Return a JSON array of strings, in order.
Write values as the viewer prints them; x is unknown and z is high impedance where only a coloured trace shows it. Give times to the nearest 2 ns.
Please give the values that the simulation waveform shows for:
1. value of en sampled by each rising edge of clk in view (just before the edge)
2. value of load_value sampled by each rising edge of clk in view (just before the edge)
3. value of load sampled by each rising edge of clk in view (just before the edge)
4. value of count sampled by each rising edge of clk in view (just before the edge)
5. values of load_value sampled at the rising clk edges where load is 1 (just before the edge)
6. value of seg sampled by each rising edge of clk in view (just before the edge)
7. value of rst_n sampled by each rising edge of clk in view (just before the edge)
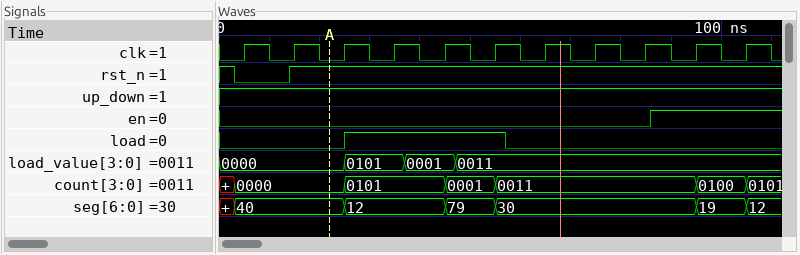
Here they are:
["0 0 0 0 0 0 0 0 0 1 1", "0000, 0000, 0000, 0101, 0001, 0011, 0011, 0011, 0011, 0011, 0011", "0 0 0 1 1 1 0 0 0 0 0", "0000, 0000, 0000, 0101, 0101, 0001, 0011, 0011, 0011, 0011, 0100", "0101, 0001, 0011", "40, 40, 40, 12, 12, 79, 30, 30, 30, 30, 19", "0 1 1 1 1 1 1 1 1 1 1"]
